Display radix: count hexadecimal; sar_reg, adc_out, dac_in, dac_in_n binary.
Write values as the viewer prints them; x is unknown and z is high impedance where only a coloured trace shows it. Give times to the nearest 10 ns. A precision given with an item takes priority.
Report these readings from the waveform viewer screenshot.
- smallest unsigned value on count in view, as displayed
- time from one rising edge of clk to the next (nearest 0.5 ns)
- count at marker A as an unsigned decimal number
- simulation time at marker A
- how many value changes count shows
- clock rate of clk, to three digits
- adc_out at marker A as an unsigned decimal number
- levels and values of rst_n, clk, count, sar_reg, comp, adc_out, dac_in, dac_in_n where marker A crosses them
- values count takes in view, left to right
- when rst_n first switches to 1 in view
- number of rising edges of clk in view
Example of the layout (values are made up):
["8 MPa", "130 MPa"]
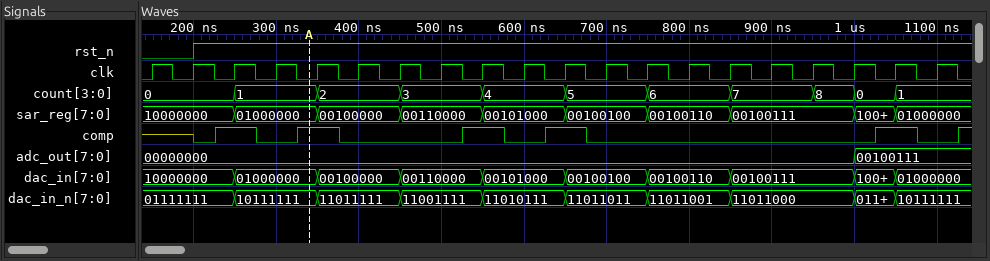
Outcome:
["0", "50 ns", "1", "340 ns", "10", "20.0 MHz", "0", "rst_n=1, clk=0, count=1, sar_reg=01000000, comp=1, adc_out=00000000, dac_in=01000000, dac_in_n=10111111", "0, 1, 2, 3, 4, 5, 6, 7, 8, 0, 1", "200 ns", "20"]
